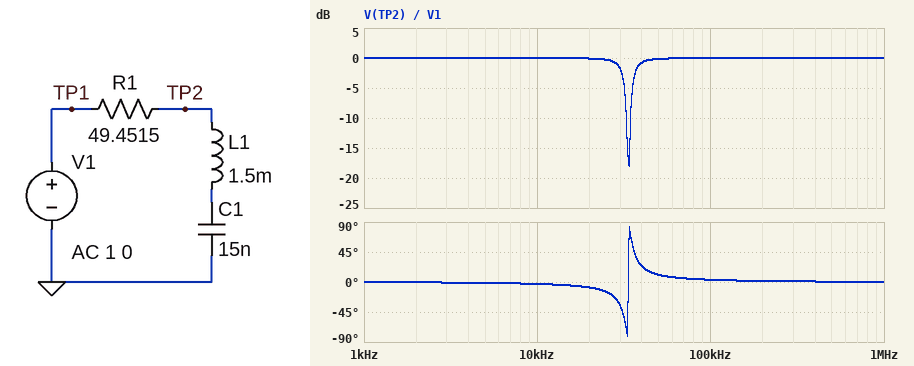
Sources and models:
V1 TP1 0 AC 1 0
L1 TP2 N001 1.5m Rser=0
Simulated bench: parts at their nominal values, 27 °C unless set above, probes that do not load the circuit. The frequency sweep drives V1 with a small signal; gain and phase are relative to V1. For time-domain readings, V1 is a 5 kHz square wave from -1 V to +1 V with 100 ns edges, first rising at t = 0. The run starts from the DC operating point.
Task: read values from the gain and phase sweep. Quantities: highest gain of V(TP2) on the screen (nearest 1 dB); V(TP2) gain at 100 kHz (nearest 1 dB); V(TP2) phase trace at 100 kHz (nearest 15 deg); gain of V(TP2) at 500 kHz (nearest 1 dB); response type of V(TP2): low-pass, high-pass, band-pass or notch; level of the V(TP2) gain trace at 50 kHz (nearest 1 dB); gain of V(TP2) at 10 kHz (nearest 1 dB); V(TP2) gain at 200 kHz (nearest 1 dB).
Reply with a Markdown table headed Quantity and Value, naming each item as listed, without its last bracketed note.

| Quantity | Value |
|---|---|
| highest gain of V(TP2) on the screen | 0 dB |
| V(TP2) gain at 100 kHz | 0 dB |
| V(TP2) phase trace at 100 kHz | 0 deg |
| gain of V(TP2) at 500 kHz | 0 dB |
| response type of V(TP2): low-pass, high-pass, band-pass or notch | notch |
| level of the V(TP2) gain trace at 50 kHz | 0 dB |
| gain of V(TP2) at 10 kHz | 0 dB |
| V(TP2) gain at 200 kHz | 0 dB |
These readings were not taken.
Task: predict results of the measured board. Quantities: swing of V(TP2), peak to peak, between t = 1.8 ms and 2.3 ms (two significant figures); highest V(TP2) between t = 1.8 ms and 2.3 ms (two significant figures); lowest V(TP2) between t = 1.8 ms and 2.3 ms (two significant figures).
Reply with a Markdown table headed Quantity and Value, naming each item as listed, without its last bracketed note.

| Quantity | Value |
|---|---|
| swing of V(TP2), peak to peak, between t = 1.8 ms and 2.3 ms | 2.5 V |
| highest V(TP2) between t = 1.8 ms and 2.3 ms | 1.2 V |
| lowest V(TP2) between t = 1.8 ms and 2.3 ms | -1.2 V |
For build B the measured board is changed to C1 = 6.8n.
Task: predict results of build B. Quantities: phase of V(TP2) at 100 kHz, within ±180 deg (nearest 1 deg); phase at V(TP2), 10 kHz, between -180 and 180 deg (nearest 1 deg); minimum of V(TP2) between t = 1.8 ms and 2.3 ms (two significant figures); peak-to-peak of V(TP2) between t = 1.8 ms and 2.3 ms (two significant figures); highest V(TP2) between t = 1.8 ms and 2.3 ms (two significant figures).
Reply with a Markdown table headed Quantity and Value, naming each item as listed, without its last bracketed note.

| Quantity | Value |
|---|---|
| phase of V(TP2) at 100 kHz, within ±180 deg | 4 deg |
| phase at V(TP2), 10 kHz, between -180 and 180 deg | -1 deg |
| minimum of V(TP2) between t = 1.8 ms and 2.3 ms | -1.1 V |
| peak-to-peak of V(TP2) between t = 1.8 ms and 2.3 ms | 2.3 V |
| highest V(TP2) between t = 1.8 ms and 2.3 ms | 1.1 V |
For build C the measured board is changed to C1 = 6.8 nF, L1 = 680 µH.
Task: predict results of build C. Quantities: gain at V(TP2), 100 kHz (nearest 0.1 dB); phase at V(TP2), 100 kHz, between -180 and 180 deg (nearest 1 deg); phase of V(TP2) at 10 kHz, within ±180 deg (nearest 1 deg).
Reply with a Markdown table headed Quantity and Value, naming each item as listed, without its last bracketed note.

| Quantity | Value |
|---|---|
| gain at V(TP2), 100 kHz | -0.3 dB |
| phase at V(TP2), 100 kHz, between -180 and 180 deg | 14 deg |
| phase of V(TP2) at 10 kHz, within ±180 deg | -1 deg |
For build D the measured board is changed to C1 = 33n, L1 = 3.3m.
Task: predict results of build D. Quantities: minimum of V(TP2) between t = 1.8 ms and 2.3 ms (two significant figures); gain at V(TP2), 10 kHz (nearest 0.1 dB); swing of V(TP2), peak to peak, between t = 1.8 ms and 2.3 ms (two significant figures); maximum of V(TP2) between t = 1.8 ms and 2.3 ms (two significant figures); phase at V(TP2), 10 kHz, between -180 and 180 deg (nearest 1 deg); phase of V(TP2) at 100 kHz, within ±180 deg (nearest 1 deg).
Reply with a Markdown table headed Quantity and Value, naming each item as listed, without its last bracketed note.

| Quantity | Value |
|---|---|
| minimum of V(TP2) between t = 1.8 ms and 2.3 ms | -1.4 V |
| gain at V(TP2), 10 kHz | -0.1 dB |
| swing of V(TP2), peak to peak, between t = 1.8 ms and 2.3 ms | 2.8 V |
| maximum of V(TP2) between t = 1.8 ms and 2.3 ms | 1.4 V |
| phase at V(TP2), 10 kHz, between -180 and 180 deg | -10 deg |
| phase of V(TP2) at 100 kHz, within ±180 deg | 1 deg |
